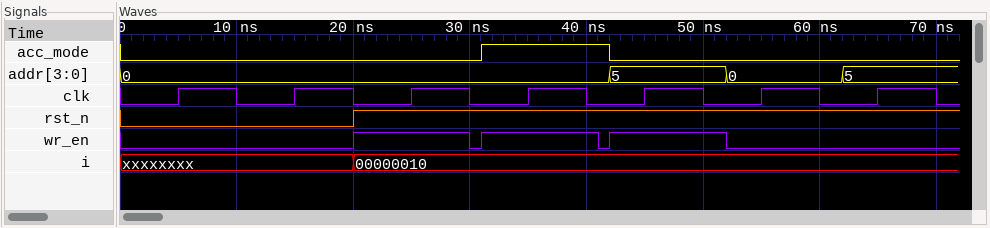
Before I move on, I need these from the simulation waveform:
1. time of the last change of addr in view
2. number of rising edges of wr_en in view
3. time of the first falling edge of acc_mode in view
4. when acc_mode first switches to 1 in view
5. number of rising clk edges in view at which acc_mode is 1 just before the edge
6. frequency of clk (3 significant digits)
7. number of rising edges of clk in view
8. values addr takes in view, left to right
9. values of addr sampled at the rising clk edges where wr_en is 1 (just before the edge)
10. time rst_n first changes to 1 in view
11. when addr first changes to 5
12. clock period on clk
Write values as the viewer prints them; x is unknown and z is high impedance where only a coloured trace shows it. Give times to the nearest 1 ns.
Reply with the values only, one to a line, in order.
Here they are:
62 ns
3
42 ns
31 ns
1
100 MHz
7
0, 5, 0, 5
0, 0, 5
20 ns
42 ns
10 ns
